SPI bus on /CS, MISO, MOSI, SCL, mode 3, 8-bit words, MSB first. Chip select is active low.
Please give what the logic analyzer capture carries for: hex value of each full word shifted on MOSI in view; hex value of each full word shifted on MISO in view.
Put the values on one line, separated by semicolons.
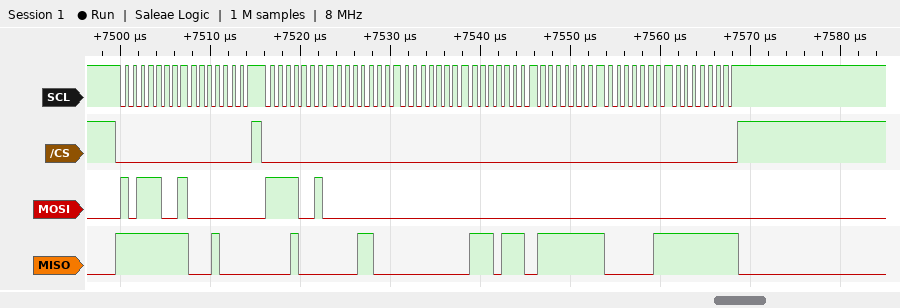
B9, 00, F2, 00, 00, 00, 00, 00, 00; FF, 10, 10, 18, 00, EE, FF, 03, FF
